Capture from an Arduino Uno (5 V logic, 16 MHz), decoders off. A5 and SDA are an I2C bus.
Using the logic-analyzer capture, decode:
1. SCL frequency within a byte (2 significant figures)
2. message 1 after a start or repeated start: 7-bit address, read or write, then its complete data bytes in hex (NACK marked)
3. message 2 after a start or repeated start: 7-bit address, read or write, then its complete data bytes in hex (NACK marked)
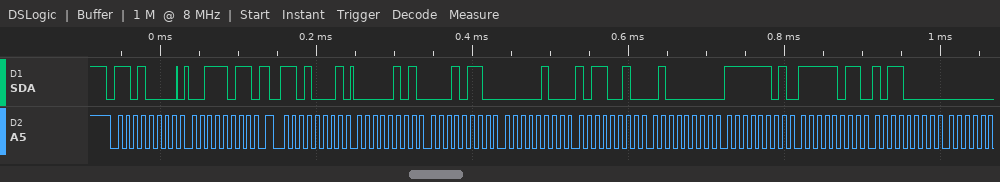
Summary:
100 kHz
0x68 write: 3B
0x68 read: 05 16 04 B2 40 FD FB B0
